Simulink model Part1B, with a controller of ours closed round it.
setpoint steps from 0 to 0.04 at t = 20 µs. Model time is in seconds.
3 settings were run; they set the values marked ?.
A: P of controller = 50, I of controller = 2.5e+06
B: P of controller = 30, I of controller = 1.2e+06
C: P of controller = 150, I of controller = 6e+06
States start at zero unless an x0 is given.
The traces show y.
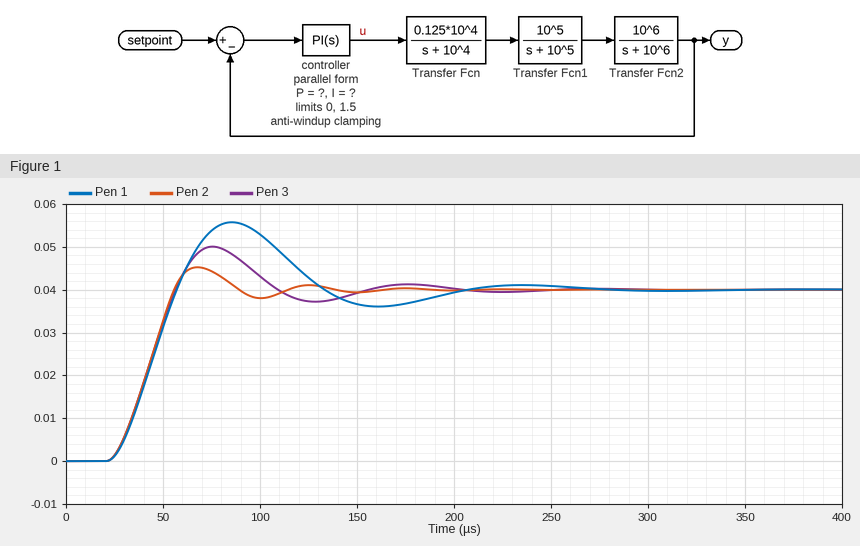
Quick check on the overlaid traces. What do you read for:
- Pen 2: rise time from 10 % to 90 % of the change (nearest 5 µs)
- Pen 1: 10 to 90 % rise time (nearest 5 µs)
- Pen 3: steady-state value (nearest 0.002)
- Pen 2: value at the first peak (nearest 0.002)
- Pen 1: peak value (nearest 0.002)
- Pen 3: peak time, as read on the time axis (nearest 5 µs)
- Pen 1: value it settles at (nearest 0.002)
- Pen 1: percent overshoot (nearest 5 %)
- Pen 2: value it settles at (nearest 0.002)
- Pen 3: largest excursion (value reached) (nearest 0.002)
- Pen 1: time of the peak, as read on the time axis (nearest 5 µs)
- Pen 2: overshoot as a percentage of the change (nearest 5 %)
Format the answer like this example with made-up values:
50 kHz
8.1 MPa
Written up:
25 µs
25 µs
0.040
0.046
0.056
75 µs
0.040
40 %
0.040
0.050
85 µs
15 %
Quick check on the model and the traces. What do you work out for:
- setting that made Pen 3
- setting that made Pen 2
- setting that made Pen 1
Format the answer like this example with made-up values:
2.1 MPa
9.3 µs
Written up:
A
C
B
